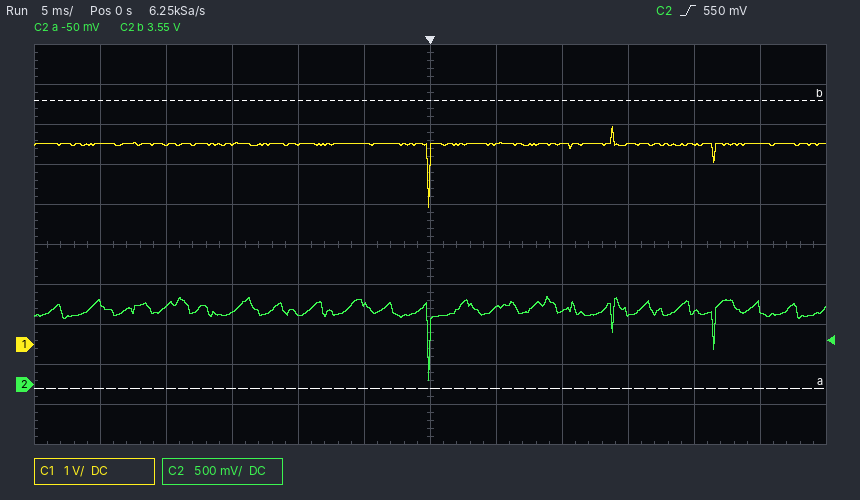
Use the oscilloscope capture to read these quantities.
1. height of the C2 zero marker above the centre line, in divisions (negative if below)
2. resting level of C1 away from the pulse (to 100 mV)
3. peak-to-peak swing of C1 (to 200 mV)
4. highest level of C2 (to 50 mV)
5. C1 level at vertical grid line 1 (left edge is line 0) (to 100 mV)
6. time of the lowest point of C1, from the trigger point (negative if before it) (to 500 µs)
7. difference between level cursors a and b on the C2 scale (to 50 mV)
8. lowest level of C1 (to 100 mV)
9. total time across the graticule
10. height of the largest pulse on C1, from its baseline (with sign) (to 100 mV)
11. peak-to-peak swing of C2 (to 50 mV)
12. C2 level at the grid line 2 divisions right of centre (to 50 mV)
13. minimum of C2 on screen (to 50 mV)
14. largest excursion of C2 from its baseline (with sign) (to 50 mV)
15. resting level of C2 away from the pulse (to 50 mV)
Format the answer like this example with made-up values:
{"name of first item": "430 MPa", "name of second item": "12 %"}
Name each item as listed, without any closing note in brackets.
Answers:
{"height of the C2 zero marker above the centre line, in divisions": "-3.5 div", "resting level of C1 away from the pulse": "5.0 V", "peak-to-peak swing of C1": "2.0 V", "highest level of C2": "1.10 V", "C1 level at vertical grid line 1 (left edge is line 0)": "5.0 V", "time of the lowest point of C1, from the trigger point (negative if before it)": "0.0 ms", "difference between level cursors a and b on the C2 scale": "3.60 V", "lowest level of C1": "3.4 V", "total time across the graticule": "60 ms", "height of the largest pulse on C1, from its baseline (with sign)": "-1.6 V", "peak-to-peak swing of C2": "1.05 V", "C2 level at the grid line 2 divisions right of centre": "900 mV", "minimum of C2 on screen": "50 mV", "largest excursion of C2 from its baseline (with sign)": "-850 mV", "resting level of C2 away from the pulse": "900 mV"}
